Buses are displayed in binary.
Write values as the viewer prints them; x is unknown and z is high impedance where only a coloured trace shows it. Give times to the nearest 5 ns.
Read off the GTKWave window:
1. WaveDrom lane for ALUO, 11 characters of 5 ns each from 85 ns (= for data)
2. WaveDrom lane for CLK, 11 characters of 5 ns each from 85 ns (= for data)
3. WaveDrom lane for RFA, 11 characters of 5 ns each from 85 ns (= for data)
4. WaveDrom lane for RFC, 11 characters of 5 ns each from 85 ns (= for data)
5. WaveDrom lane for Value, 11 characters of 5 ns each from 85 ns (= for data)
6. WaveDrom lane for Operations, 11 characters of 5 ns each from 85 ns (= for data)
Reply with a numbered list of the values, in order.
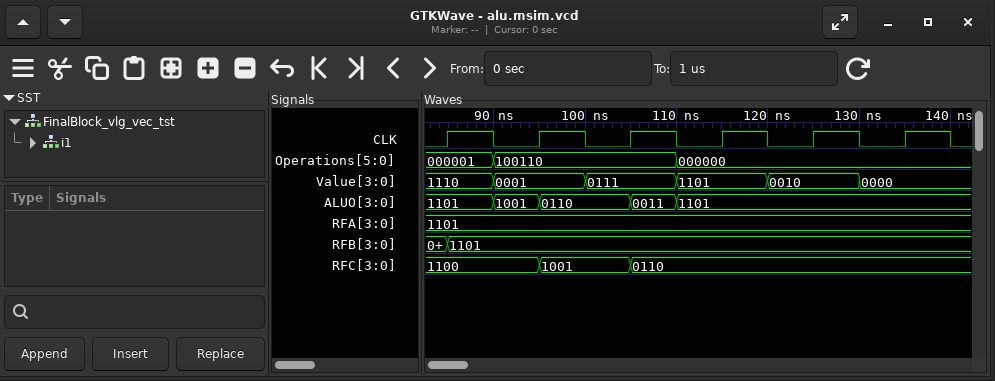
1. {name: 'ALUO', wave: '===.==.....', data: '1101 1001 0110 0011 1101'}
2. {name: 'CLK', wave: '10101010101'}
3. {name: 'RFA', wave: '=..........', data: '1101'}
4. {name: 'RFC', wave: '=.=.=......', data: '1100 1001 0110'}
5. {name: 'Value', wave: '==.=.=.=.=.', data: '1110 0001 0111 1101 0010 0000'}
6. {name: 'Operations', wave: '==...=.....', data: '000001 100110 000000'}
